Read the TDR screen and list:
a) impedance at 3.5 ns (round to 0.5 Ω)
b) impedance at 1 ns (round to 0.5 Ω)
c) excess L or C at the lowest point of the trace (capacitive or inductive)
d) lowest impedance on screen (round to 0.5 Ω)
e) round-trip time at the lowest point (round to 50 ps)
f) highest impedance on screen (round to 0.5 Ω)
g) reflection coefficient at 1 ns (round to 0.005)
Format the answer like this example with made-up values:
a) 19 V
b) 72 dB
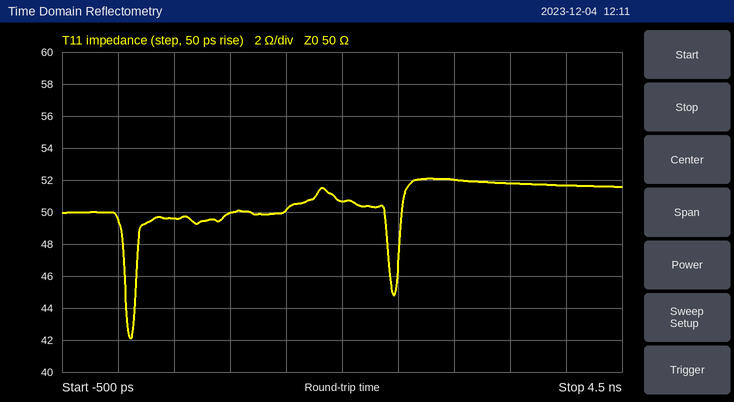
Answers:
a) 52.0 Ω
b) 50.0 Ω
c) capacitive
d) 42.0 Ω
e) 100 ps
f) 52.0 Ω
g) 0.000
